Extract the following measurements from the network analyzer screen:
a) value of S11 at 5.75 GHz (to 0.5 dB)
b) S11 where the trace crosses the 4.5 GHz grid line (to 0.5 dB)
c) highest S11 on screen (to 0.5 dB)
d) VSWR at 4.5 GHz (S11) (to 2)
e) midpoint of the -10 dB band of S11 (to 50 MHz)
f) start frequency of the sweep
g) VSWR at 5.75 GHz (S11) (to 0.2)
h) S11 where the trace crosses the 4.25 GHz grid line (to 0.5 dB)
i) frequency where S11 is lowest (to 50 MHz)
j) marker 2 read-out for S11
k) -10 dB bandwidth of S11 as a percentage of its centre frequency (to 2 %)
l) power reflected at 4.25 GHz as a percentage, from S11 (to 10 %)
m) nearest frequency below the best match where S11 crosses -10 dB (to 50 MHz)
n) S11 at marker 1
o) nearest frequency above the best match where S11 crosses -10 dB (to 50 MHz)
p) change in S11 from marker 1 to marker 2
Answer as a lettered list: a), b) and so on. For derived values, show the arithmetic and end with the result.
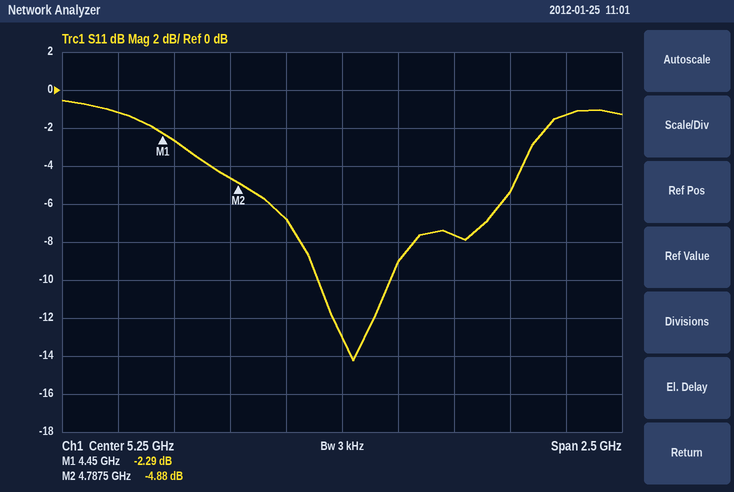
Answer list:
a) -7.5 dB
b) -2.5 dB
c) -0.5 dB
d) |Γ| = 10^(-2.5/20) = 0.7499; VSWR = (1 + 0.7499)/(1 − 0.7499) ≈ 7.00, so 6 to the nearest 2
e) 5.30 GHz
f) 4 GHz
g) |Γ| = 10^(-7.5/20) = 0.4217; VSWR = (1 + 0.4217)/(1 − 0.4217) ≈ 2.46, so 2.4 to the nearest 0.2
h) -1.0 dB
i) 5.30 GHz
j) -4.88 dB
k) 300 MHz / 5.3 GHz ≈ 6 %
l) 10^(-1/10) ≈ 79.4 %, so 80 % to the nearest 10 %
m) 5.15 GHz
n) -2.29 dB
o) 5.45 GHz
p) -4.88 − (-2.29) = -2.59 dB
